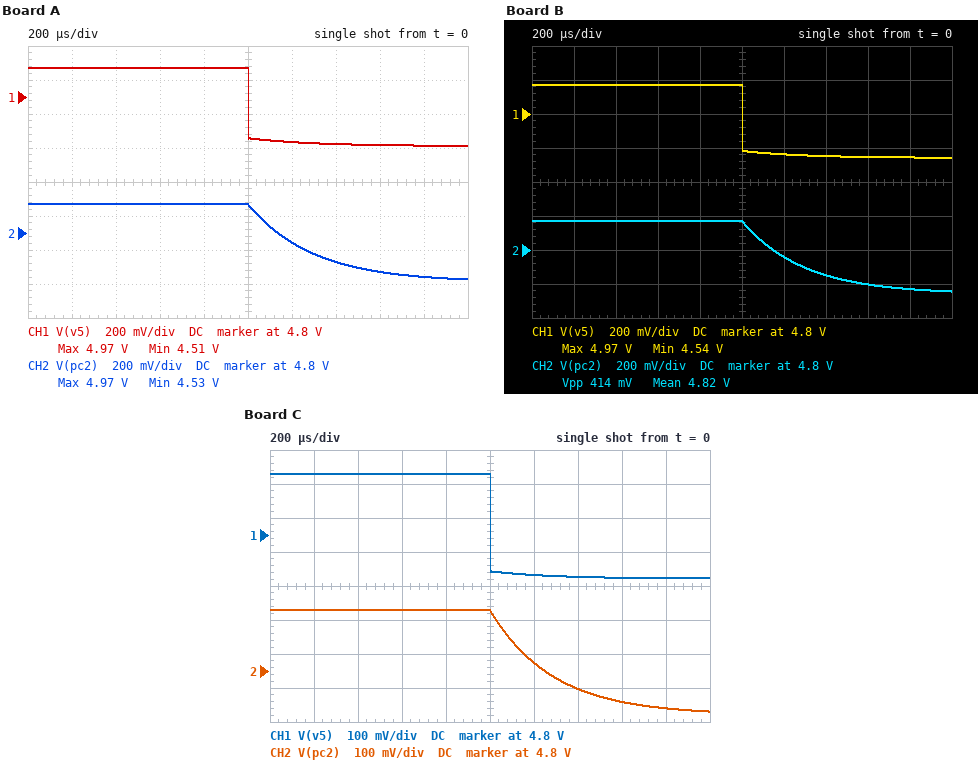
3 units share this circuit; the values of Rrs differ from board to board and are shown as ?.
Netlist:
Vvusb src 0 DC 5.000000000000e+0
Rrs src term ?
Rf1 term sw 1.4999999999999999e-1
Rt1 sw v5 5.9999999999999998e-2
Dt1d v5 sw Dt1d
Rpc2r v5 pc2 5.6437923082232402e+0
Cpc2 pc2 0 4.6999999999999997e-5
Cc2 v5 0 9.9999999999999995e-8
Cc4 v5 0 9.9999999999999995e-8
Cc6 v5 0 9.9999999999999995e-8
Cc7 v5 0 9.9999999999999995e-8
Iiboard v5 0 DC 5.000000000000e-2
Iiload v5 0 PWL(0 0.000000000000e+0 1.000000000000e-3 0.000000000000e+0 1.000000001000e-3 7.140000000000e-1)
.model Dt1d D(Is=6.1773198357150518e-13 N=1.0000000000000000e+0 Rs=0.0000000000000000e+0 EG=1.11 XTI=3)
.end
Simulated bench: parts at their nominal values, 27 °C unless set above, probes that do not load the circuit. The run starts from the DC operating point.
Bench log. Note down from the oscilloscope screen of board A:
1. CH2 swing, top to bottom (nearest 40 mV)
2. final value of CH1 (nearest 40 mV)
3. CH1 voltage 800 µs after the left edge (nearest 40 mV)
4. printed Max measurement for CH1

440 mV
4.52 V
4.96 V
4.97 V
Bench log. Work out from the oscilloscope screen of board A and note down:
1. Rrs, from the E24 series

0.43 Ω
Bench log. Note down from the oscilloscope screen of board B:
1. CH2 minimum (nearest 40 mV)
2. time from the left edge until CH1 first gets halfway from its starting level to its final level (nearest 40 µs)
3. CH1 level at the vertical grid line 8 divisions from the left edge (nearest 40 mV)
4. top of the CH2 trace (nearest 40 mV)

4.56 V
1.00 ms
4.56 V
4.96 V
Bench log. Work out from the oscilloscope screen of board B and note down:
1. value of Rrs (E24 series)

0.39 Ω
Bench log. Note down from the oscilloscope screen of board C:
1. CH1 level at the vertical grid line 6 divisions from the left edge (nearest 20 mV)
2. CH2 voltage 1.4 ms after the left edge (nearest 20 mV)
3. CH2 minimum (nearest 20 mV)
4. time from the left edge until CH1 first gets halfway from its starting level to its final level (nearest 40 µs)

4.68 V
4.74 V
4.68 V
1.00 ms
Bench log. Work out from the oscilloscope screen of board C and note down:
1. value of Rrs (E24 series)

0.22 Ω
